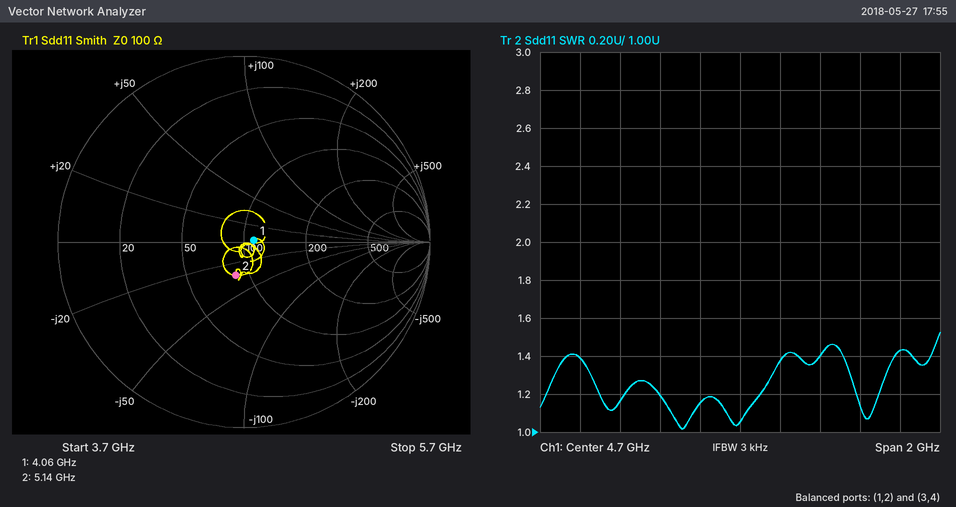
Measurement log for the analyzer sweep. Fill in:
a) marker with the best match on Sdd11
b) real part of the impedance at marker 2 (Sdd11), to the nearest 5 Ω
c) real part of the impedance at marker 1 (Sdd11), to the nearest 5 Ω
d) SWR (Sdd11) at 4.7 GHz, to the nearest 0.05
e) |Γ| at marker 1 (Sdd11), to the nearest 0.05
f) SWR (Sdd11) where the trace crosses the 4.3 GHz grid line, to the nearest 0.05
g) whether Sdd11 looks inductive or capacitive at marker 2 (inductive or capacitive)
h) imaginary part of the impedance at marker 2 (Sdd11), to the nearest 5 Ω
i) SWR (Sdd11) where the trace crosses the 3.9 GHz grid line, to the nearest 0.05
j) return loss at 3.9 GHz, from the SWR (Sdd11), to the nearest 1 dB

marker 1
85 Ω
110 Ω
1.05
0.05
1.20
capacitive
-30 Ω
1.40
16 dB
